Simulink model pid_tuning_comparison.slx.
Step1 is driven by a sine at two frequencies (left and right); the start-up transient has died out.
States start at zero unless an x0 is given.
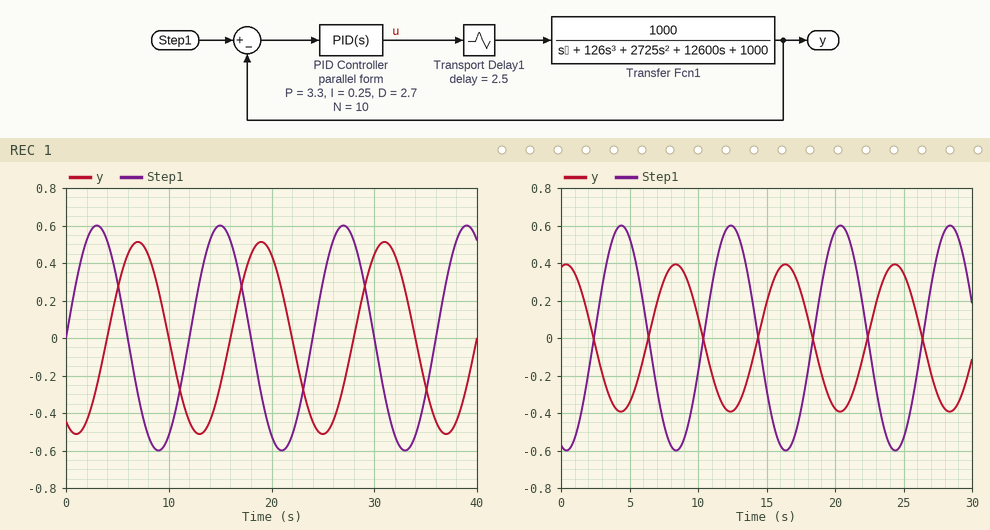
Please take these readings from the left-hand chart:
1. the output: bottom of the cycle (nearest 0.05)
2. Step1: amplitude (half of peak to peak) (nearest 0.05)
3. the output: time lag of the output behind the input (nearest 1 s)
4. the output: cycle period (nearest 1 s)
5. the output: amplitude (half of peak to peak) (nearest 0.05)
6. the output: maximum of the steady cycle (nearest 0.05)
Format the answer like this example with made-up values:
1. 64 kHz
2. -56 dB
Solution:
1. -0.50
2. 0.60
3. 4 s
4. 12 s
5. 0.50
6. 0.50
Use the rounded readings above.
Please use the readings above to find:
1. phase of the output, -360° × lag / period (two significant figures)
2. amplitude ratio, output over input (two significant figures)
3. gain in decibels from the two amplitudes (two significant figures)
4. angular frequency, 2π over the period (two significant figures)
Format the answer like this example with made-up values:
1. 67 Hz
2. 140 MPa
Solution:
1. -120°
2. 0.83
3. -1.6 dB
4. 0.52 rad/s
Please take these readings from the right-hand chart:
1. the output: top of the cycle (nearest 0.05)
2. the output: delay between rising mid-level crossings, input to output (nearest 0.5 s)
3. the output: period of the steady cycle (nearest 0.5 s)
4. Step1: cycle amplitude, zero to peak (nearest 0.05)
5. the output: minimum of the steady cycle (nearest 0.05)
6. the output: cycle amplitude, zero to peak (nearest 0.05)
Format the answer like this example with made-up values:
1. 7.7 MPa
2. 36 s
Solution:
1. 0.40
2. 4.0 s
3. 8.0 s
4. 0.60
5. -0.40
6. 0.40
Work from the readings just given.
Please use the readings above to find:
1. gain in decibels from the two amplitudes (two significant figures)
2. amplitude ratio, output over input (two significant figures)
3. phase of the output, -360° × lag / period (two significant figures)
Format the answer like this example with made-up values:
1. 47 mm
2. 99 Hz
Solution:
1. -3.5 dB
2. 0.67
3. -180°
